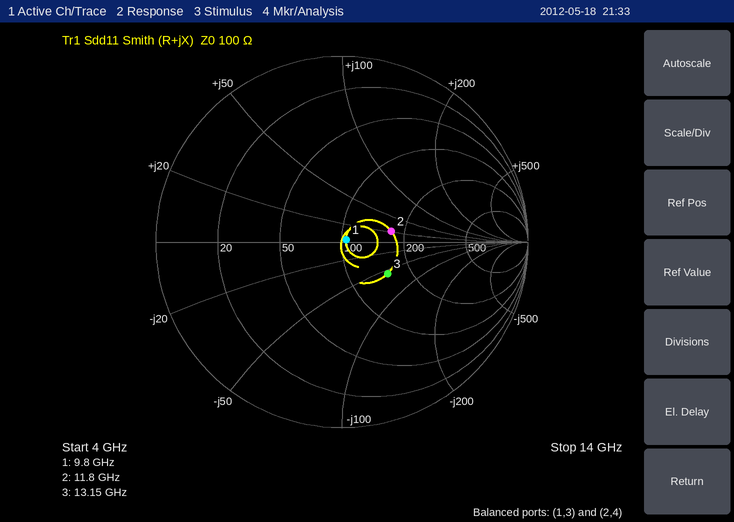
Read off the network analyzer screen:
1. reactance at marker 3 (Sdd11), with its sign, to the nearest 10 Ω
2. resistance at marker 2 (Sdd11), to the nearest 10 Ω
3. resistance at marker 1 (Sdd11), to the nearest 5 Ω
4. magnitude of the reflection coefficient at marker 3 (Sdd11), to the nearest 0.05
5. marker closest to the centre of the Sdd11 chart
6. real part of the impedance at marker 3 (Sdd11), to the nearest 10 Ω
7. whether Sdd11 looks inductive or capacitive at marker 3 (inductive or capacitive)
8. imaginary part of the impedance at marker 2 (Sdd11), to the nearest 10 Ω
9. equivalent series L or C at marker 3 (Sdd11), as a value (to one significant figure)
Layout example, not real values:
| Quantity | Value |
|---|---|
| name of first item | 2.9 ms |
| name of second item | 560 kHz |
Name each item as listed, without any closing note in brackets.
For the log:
| Quantity | Value |
|---|---|
| reactance at marker 3 (Sdd11), with its sign, to the nearest 10 Ω | -60 Ω |
| resistance at marker 2 (Sdd11), to the nearest 10 Ω | 170 Ω |
| resistance at marker 1 (Sdd11), to the nearest 5 Ω | 105 Ω |
| magnitude of the reflection coefficient at marker 3 (Sdd11), to the nearest 0.05 | 0.30 |
| marker closest to the centre of the Sdd11 chart | marker 1 |
| real part of the impedance at marker 3 (Sdd11), to the nearest 10 Ω | 150 Ω |
| whether Sdd11 looks inductive or capacitive at marker 3 | capacitive |
| imaginary part of the impedance at marker 2 (Sdd11), to the nearest 10 Ω | +20 Ω |
| equivalent series L or C at marker 3 (Sdd11), as a value | 200 fF |
